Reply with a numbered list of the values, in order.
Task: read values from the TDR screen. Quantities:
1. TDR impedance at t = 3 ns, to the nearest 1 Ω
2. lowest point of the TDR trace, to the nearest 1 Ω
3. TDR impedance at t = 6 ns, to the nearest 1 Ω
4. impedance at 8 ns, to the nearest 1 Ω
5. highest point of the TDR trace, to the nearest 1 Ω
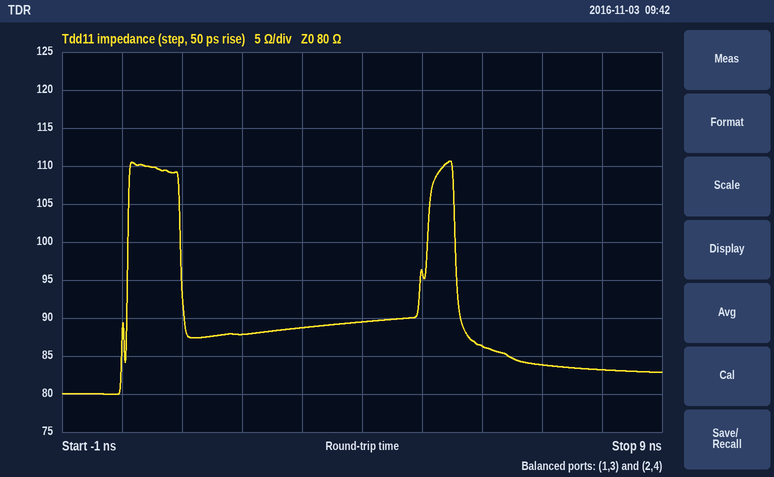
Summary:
1. 89 Ω
2. 80 Ω
3. 86 Ω
4. 83 Ω
5. 111 Ω
